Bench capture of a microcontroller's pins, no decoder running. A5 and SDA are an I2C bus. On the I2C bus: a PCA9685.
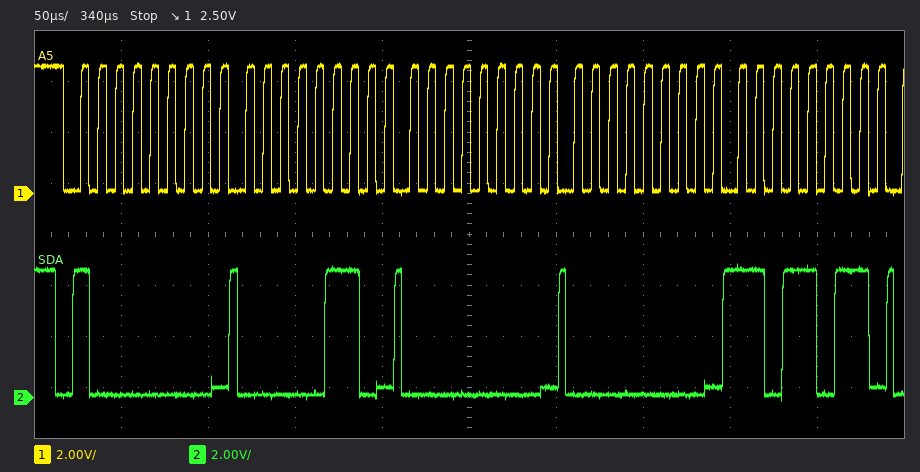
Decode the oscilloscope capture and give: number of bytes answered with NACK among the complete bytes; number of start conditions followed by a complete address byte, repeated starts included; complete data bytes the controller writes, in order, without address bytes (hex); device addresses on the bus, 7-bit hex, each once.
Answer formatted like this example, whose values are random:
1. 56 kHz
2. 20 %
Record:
1. 0
2. 1
3. 06 00 00 DB
4. 0x40
